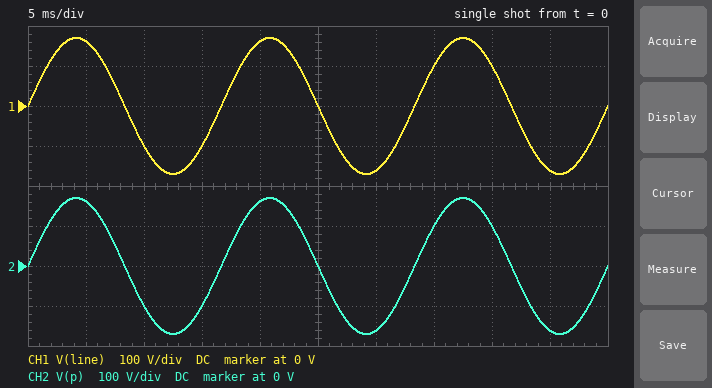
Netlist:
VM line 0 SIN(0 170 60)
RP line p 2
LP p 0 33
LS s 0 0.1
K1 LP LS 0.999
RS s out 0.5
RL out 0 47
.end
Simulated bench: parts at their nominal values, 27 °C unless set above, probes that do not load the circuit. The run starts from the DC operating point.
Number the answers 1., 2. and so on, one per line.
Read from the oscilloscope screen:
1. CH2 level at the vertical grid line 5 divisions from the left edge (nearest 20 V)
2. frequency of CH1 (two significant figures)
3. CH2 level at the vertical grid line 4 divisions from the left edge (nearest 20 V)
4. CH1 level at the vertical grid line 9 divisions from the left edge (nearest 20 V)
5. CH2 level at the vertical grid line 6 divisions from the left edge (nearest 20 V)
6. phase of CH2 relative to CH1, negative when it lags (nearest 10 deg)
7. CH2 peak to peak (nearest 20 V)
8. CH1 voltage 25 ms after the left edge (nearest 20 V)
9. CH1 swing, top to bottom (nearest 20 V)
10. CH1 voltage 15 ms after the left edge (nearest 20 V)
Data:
1. 0 V
2. 60 Hz
3. 160 V
4. -160 V
5. -160 V
6. 0 deg
7. 340 V
8. 0 V
9. 340 V
10. -100 V
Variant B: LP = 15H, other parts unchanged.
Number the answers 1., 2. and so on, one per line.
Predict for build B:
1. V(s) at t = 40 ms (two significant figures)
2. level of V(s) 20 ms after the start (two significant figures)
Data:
1. 8.2 V
2. 13 V
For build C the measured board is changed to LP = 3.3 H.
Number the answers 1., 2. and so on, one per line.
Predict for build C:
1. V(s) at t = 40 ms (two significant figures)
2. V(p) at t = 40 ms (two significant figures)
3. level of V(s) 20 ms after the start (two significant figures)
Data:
1. 17 V
2. 99 V
3. 28 V
